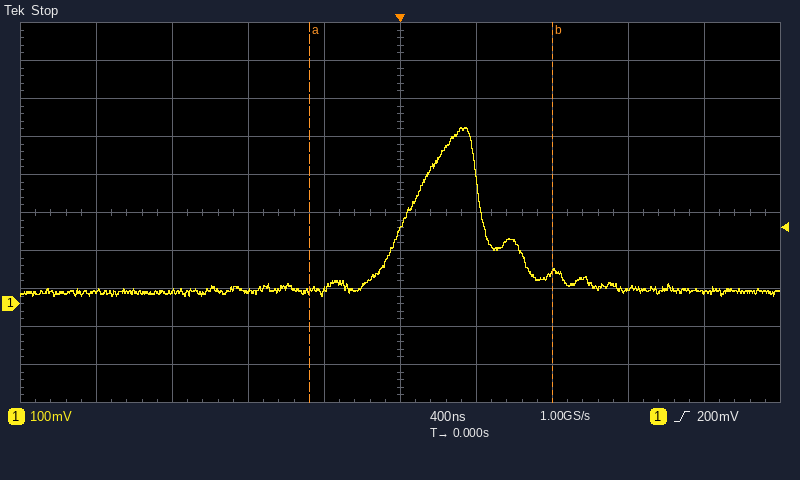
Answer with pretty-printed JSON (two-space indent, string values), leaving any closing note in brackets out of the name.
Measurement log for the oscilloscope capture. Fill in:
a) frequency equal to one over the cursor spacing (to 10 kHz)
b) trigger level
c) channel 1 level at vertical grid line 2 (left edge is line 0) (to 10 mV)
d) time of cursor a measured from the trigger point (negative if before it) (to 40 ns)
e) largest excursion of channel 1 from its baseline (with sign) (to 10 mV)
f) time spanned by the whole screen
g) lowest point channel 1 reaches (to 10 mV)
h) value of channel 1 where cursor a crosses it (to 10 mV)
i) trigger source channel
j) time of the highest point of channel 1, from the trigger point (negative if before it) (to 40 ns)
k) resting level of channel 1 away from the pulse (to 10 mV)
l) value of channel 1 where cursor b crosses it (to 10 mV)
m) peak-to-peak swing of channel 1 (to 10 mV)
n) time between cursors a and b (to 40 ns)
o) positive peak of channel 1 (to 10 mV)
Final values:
{
  "frequency equal to one over the cursor spacing": "780 kHz",
  "trigger level": "200 mV",
  "channel 1 level at vertical grid line 2 (left edge is line 0)": "30 mV",
  "time of cursor a measured from the trigger point (negative if before it)": "-480 ns",
  "largest excursion of channel 1 from its baseline (with sign)": "+430 mV",
  "time spanned by the whole screen": "4 µs",
  "lowest point channel 1 reaches": "20 mV",
  "value of channel 1 where cursor a crosses it": "30 mV",
  "trigger source channel": "channel 1",
  "time of the highest point of channel 1, from the trigger point (negative if before it)": "+320 ns",
  "resting level of channel 1 away from the pulse": "30 mV",
  "value of channel 1 where cursor b crosses it": "80 mV",
  "peak-to-peak swing of channel 1": "440 mV",
  "time between cursors a and b": "1.28 µs",
  "positive peak of channel 1": "460 mV"
}
